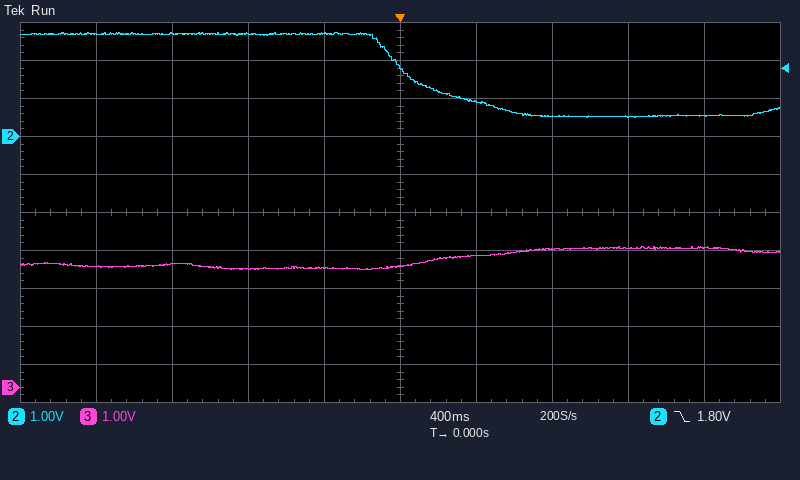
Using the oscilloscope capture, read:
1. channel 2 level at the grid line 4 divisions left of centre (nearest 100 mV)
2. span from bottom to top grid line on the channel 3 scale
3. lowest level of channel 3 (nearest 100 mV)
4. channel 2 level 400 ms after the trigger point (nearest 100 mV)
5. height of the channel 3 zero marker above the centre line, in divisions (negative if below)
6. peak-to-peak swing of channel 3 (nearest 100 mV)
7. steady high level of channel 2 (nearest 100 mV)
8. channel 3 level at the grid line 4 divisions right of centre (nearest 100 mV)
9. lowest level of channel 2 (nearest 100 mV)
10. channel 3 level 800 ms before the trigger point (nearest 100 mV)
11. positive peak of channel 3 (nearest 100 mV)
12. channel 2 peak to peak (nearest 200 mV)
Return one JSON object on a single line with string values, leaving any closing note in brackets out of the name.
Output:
{"channel 2 level at the grid line 4 divisions left of centre": "2.7 V", "span from bottom to top grid line on the channel 3 scale": "10 V", "lowest level of channel 3": "3.1 V", "channel 2 level 400 ms after the trigger point": "900 mV", "height of the channel 3 zero marker above the centre line, in divisions": "-4.6 div", "peak-to-peak swing of channel 3": "600 mV", "steady high level of channel 2": "2.7 V", "channel 3 level at the grid line 4 divisions right of centre": "3.7 V", "lowest level of channel 2": "500 mV", "channel 3 level 800 ms before the trigger point": "3.1 V", "positive peak of channel 3": "3.7 V", "channel 2 peak to peak": "2.2 V"}
